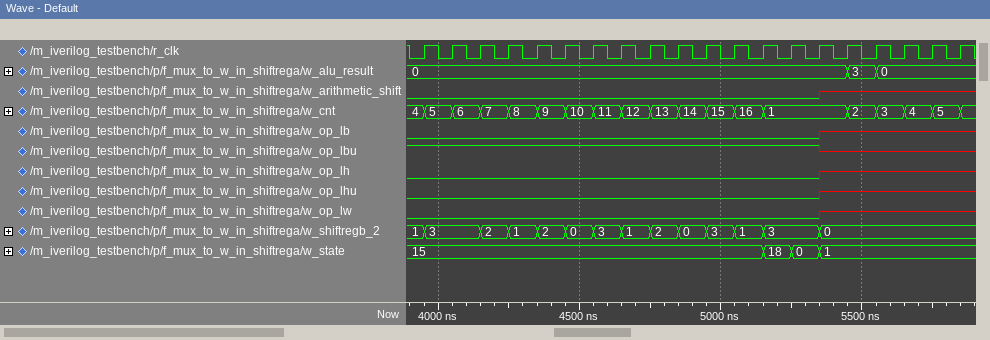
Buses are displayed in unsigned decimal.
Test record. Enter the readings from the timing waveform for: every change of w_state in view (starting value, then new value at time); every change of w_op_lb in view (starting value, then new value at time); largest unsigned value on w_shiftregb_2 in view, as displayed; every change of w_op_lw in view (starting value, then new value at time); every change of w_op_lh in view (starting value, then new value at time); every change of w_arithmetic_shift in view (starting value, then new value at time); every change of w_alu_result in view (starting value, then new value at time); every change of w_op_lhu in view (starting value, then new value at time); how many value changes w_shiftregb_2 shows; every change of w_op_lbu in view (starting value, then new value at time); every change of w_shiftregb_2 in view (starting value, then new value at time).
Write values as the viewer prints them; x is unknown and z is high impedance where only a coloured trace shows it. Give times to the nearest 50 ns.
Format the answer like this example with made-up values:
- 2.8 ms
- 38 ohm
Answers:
- 15, 18 at 5150 ns, 0 at 5250 ns, 1 at 5350 ns
- 0, x at 5350 ns
- 3
- 0, x at 5350 ns
- 0, x at 5350 ns
- 0, x at 5350 ns
- 0, 3 at 5450 ns, 0 at 5550 ns
- 0, x at 5350 ns
- 13
- 1, x at 5350 ns
- 1, 3 at 3950 ns, 2 at 4150 ns, 1 at 4250 ns, 2 at 4350 ns, 0 at 4450 ns, 3 at 4550 ns, 1 at 4650 ns, 2 at 4750 ns, 0 at 4850 ns, 3 at 4950 ns, 1 at 5050 ns, 3 at 5150 ns, 0 at 5350 ns
